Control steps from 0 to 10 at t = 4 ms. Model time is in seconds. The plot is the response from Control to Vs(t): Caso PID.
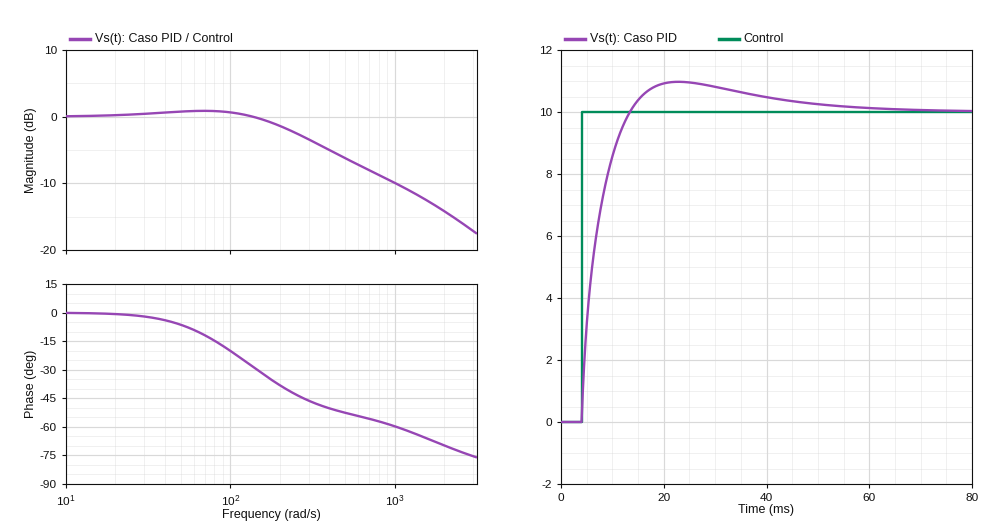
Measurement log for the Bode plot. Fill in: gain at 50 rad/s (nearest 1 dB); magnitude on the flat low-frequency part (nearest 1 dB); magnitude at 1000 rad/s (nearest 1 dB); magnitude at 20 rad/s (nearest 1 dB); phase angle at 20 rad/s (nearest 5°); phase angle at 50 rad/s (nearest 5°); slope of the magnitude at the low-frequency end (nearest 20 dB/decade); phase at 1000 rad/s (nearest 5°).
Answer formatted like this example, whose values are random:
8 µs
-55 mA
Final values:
1 dB
0 dB
-10 dB
0 dB
0°
-5°
0 dB/decade
-60°
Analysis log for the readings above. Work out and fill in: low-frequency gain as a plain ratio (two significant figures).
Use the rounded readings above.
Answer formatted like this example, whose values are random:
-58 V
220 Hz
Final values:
1.0
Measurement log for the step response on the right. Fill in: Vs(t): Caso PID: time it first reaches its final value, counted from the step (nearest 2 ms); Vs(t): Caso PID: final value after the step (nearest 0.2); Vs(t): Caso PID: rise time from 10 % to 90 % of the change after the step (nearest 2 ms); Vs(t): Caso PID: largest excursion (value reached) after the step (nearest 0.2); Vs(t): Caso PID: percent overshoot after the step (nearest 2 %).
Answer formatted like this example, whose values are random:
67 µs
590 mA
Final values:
10 ms
10.0
6 ms
11.0
10 %
